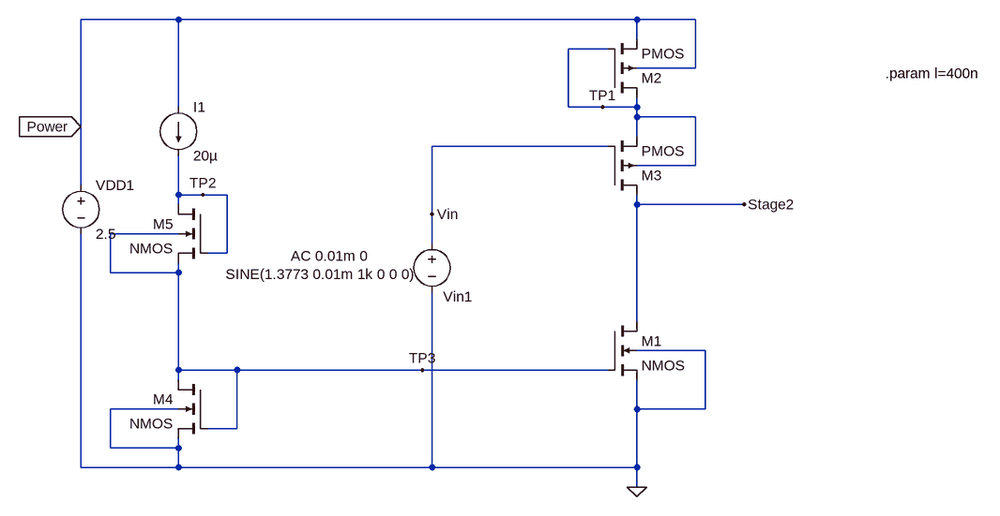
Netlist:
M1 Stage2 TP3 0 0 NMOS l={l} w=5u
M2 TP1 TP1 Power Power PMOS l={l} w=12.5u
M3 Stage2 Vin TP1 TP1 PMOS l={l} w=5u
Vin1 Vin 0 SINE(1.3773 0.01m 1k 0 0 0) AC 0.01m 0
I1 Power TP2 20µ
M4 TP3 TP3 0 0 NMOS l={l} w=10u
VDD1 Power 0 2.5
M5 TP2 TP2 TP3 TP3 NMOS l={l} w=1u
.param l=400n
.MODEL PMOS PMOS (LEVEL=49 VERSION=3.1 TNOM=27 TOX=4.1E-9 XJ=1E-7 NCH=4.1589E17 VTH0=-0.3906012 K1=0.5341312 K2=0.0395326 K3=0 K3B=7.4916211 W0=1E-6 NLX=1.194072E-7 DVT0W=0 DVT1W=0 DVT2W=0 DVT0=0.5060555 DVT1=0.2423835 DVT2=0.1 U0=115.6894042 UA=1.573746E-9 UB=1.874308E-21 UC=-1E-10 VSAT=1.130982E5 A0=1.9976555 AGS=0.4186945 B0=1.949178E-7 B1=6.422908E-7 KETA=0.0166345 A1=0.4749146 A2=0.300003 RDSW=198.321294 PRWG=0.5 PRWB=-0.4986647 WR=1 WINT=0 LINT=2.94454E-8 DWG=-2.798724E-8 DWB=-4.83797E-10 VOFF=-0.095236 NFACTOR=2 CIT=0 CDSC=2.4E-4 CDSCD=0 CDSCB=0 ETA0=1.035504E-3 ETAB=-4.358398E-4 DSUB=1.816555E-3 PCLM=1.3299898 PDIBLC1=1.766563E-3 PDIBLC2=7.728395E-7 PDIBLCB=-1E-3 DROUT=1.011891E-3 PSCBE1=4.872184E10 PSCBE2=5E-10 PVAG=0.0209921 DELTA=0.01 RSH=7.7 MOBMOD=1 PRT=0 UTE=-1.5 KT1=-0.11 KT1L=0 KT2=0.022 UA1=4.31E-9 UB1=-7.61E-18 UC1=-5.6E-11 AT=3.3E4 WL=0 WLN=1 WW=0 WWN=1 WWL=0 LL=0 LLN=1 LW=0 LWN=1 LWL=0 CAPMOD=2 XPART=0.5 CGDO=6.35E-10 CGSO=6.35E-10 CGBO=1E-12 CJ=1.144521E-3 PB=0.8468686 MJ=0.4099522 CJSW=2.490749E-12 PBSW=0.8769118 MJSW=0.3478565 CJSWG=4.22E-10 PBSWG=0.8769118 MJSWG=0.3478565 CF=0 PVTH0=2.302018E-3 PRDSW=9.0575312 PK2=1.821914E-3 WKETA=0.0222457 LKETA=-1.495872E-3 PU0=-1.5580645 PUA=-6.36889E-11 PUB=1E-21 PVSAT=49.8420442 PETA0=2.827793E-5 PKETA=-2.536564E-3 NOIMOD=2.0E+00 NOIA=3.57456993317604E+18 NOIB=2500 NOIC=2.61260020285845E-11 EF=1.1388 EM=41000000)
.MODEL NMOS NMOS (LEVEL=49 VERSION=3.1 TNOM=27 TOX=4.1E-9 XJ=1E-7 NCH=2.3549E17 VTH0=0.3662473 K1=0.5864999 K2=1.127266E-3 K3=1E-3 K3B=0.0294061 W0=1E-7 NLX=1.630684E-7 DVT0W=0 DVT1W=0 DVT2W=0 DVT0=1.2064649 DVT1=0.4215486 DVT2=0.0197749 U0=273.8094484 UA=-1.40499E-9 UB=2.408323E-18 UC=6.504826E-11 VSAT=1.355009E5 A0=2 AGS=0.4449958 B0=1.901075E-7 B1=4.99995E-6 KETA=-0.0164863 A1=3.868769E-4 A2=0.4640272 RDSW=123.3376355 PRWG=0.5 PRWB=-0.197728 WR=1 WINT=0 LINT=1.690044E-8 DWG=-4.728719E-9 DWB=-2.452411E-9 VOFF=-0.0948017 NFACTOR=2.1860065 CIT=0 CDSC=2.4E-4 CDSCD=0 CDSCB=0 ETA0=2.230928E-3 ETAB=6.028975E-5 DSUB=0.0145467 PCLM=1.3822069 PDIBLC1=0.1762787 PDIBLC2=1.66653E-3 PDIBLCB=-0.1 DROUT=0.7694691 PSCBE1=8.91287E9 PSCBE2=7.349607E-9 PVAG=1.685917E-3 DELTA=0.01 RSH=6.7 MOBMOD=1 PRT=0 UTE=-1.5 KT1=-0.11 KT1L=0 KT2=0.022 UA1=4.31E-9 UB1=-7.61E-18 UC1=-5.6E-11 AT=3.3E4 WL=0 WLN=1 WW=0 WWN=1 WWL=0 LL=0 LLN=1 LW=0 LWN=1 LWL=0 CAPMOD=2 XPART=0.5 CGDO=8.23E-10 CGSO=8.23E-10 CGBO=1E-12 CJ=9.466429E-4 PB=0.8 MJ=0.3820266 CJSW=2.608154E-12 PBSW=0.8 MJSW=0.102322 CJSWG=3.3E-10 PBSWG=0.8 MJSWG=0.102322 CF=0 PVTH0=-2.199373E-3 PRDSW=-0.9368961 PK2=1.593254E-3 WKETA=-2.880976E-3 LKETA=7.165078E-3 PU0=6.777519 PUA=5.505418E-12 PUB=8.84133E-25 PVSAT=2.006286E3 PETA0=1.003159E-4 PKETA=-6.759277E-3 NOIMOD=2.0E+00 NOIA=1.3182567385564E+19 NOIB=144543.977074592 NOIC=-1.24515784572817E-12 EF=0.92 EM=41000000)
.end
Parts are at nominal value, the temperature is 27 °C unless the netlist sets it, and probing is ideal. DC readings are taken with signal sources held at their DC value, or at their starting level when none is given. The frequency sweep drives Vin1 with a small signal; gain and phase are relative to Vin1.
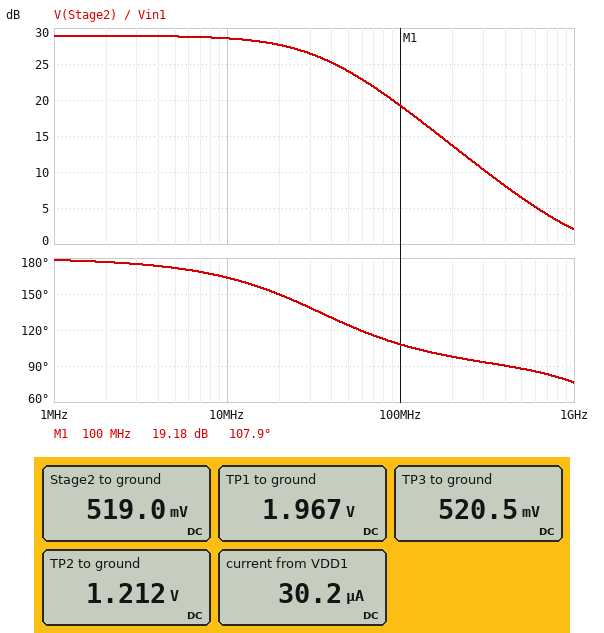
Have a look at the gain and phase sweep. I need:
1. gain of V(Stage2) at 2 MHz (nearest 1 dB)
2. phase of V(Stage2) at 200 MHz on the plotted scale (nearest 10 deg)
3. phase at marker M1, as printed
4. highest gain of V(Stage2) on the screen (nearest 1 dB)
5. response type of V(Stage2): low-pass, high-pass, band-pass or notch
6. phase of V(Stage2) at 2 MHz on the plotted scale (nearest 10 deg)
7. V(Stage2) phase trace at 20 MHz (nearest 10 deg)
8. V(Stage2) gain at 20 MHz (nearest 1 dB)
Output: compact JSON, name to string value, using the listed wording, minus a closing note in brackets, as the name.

{"gain of V(Stage2) at 2 MHz": "29 dB", "phase of V(Stage2) at 200 MHz on the plotted scale": "100 deg", "phase at marker M1, as printed": "107.9 deg", "highest gain of V(Stage2) on the screen": "29 dB", "response type of V(Stage2): low-pass, high-pass, band-pass or notch": "low-pass", "phase of V(Stage2) at 2 MHz on the plotted scale": "180 deg", "V(Stage2) phase trace at 20 MHz": "150 deg", "V(Stage2) gain at 20 MHz": "28 dB"}
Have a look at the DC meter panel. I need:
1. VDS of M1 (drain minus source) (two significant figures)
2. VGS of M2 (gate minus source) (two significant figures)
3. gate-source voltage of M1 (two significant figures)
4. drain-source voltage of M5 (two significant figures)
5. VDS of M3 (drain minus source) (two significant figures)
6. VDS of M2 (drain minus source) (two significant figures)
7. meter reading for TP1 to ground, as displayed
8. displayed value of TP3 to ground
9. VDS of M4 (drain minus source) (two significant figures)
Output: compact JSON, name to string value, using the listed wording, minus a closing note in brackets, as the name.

{"VDS of M1 (drain minus source)": "520 mV", "VGS of M2 (gate minus source)": "-530 mV", "gate-source voltage of M1": "520 mV", "drain-source voltage of M5": "690 mV", "VDS of M3 (drain minus source)": "-1.4 V", "VDS of M2 (drain minus source)": "-530 mV", "meter reading for TP1 to ground, as displayed": "1.967 V", "displayed value of TP3 to ground": "520.5 mV", "VDS of M4 (drain minus source)": "520 mV"}
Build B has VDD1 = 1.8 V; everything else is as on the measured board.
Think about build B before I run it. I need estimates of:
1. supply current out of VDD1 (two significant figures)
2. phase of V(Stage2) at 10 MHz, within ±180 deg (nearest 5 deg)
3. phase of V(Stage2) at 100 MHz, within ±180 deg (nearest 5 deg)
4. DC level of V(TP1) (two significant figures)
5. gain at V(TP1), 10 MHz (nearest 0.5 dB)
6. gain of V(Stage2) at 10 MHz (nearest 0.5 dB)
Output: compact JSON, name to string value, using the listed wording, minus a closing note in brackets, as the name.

{"supply current out of VDD1": "20 µA", "phase of V(Stage2) at 10 MHz, within ±180 deg": "115 deg", "phase of V(Stage2) at 100 MHz, within ±180 deg": "90 deg", "DC level of V(TP1)": "1.6 V", "gain at V(TP1), 10 MHz": "-12.5 dB", "gain of V(Stage2) at 10 MHz": "-58.5 dB"}
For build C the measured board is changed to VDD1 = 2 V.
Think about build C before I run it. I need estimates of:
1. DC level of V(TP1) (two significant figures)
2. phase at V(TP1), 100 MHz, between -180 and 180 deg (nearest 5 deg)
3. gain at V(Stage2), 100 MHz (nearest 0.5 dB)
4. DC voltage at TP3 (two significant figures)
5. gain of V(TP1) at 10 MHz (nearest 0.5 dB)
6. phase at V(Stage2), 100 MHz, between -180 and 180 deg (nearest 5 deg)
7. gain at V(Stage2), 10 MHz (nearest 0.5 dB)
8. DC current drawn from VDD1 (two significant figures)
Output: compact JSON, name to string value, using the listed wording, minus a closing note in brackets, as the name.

{"DC level of V(TP1)": "1.7 V", "phase at V(TP1), 100 MHz, between -180 and 180 deg": "-10 deg", "gain at V(Stage2), 100 MHz": "-38.0 dB", "DC voltage at TP3": "520 mV", "gain of V(TP1) at 10 MHz": "-7.5 dB", "phase at V(Stage2), 100 MHz, between -180 and 180 deg": "115 deg", "gain at V(Stage2), 10 MHz": "-47.5 dB", "DC current drawn from VDD1": "20 µA"}
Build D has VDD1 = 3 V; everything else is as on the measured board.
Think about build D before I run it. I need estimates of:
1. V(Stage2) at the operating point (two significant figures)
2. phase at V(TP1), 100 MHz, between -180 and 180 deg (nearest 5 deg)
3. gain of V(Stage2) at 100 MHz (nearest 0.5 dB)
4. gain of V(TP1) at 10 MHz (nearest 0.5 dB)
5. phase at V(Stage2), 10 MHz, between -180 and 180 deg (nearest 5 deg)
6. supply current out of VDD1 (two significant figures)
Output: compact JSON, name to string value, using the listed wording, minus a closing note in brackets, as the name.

{"V(Stage2) at the operating point": "2.4 V", "phase at V(TP1), 100 MHz, between -180 and 180 deg": "80 deg", "gain of V(Stage2) at 100 MHz": "-22.0 dB", "gain of V(TP1) at 10 MHz": "-44.0 dB", "phase at V(Stage2), 10 MHz, between -180 and 180 deg": "170 deg", "supply current out of VDD1": "34 µA"}
